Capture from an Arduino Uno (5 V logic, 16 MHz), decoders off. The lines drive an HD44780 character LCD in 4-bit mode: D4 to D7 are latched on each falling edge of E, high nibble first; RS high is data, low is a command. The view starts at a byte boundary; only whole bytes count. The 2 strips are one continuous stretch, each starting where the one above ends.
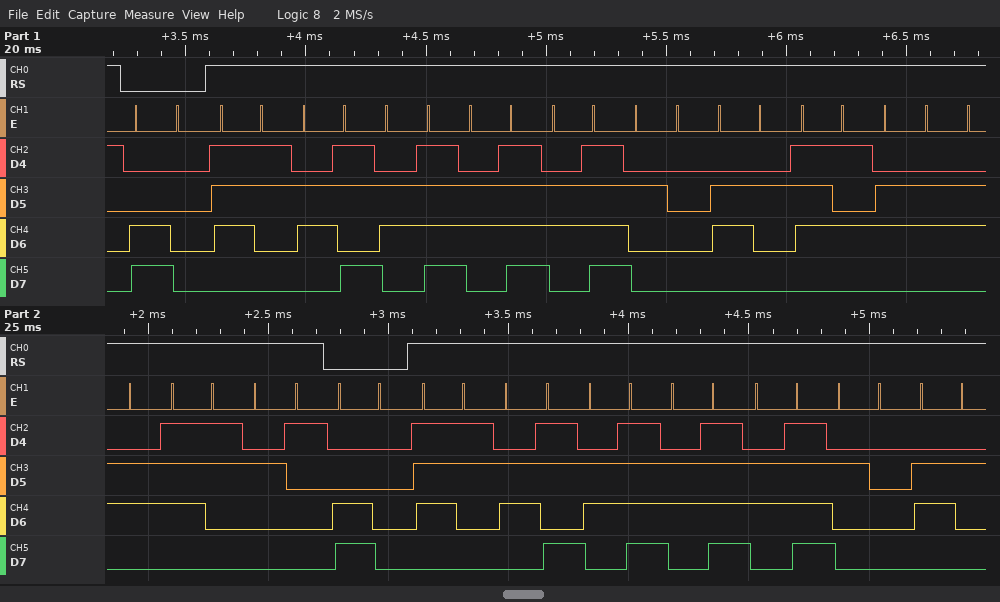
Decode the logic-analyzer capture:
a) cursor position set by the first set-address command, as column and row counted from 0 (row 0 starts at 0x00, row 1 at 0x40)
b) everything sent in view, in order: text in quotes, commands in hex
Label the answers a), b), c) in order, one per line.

a) column 0, row 1
b) 0xC0 "skooo buffs!" 0xC0 "skooo b"
